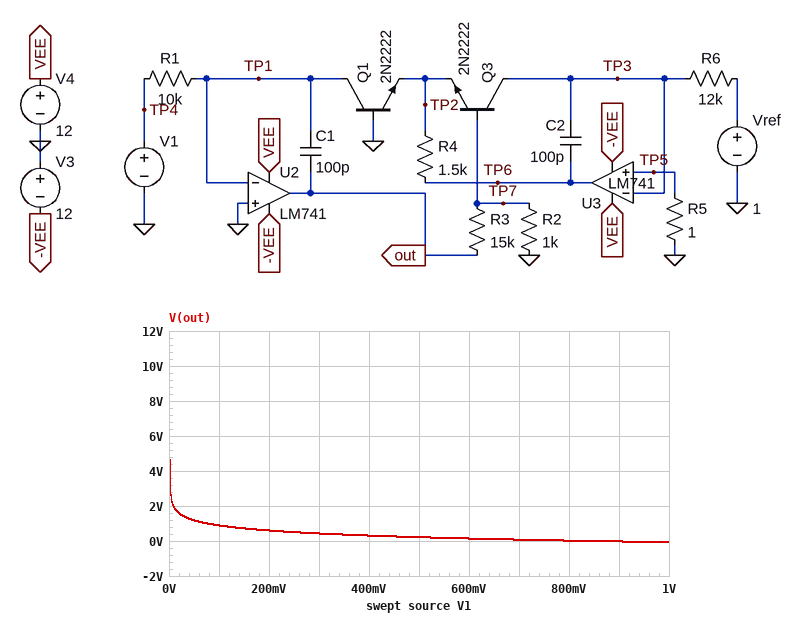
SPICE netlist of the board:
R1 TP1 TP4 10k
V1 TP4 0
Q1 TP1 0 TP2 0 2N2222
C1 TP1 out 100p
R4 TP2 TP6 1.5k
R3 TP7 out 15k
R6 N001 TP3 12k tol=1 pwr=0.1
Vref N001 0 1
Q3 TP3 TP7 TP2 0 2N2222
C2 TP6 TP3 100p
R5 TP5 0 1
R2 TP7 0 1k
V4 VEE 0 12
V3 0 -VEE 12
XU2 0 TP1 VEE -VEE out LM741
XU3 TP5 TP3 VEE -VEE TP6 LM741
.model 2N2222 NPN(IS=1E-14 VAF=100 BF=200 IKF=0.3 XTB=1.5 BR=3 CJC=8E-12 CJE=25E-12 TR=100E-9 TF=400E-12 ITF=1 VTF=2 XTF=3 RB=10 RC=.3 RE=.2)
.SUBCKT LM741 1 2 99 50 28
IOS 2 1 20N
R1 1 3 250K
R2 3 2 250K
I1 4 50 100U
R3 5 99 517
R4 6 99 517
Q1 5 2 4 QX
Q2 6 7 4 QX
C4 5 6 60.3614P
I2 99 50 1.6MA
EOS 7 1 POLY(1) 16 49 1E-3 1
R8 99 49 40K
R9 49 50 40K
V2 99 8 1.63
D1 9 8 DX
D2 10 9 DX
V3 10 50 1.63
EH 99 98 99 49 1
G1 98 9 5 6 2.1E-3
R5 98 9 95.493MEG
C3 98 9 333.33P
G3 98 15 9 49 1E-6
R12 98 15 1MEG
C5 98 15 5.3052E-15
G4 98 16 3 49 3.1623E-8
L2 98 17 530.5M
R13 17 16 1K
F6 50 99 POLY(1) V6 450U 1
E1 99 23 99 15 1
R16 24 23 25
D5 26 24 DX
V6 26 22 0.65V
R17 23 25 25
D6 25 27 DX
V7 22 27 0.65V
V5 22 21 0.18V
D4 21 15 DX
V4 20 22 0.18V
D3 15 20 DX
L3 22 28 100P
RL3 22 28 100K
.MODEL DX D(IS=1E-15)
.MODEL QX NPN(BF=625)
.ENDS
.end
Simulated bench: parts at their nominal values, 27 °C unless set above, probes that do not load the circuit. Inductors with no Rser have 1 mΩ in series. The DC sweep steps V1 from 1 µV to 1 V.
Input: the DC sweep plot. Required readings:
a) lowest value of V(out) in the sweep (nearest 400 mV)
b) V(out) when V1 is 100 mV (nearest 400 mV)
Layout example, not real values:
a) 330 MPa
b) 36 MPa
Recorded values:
a) 0 V
b) 800 mV
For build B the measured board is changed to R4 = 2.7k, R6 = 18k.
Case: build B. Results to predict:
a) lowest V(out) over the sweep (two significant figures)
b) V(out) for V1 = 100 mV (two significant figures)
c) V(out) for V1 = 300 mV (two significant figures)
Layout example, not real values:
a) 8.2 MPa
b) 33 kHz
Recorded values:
a) -240 mV
b) 720 mV
c) 260 mV
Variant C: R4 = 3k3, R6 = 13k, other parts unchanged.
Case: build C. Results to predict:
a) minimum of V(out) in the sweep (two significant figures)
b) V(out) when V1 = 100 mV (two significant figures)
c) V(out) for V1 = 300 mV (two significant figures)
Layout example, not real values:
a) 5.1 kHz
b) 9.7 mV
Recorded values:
a) -100 mV
b) 860 mV
c) 400 mV
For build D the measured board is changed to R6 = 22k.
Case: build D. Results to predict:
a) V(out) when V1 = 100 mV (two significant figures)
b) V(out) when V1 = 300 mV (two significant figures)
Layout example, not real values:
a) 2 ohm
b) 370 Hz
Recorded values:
a) 640 mV
b) 180 mV
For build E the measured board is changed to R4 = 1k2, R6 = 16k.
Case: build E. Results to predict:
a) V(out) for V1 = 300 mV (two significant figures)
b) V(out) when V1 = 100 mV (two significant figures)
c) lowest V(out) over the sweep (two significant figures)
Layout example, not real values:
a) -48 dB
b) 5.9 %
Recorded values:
a) 310 mV
b) 770 mV
c) -190 mV
